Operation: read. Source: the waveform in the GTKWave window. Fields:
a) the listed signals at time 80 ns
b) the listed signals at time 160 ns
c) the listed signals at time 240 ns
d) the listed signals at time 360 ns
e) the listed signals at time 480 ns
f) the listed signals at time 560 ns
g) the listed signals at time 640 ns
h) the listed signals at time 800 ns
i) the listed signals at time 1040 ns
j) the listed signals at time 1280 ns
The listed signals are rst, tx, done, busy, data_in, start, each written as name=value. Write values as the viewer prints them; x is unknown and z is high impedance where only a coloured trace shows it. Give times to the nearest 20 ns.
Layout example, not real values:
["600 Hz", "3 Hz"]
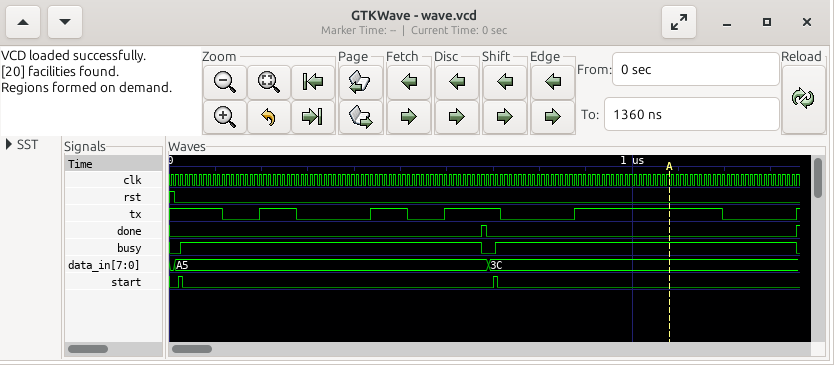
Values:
["rst=0, tx=1, done=0, busy=1, data_in=A5, start=0", "rst=0, tx=0, done=0, busy=1, data_in=A5, start=0", "rst=0, tx=1, done=0, busy=1, data_in=A5, start=0", "rst=0, tx=0, done=0, busy=1, data_in=A5, start=0", "rst=0, tx=1, done=0, busy=1, data_in=A5, start=0", "rst=0, tx=0, done=0, busy=1, data_in=A5, start=0", "rst=0, tx=1, done=0, busy=1, data_in=A5, start=0", "rst=0, tx=0, done=0, busy=1, data_in=3C, start=0", "rst=0, tx=1, done=0, busy=1, data_in=3C, start=0", "rst=0, tx=0, done=0, busy=1, data_in=3C, start=0"]
